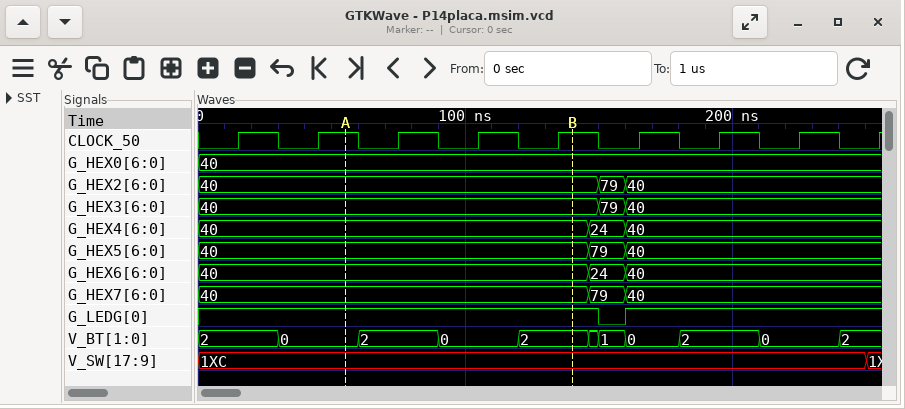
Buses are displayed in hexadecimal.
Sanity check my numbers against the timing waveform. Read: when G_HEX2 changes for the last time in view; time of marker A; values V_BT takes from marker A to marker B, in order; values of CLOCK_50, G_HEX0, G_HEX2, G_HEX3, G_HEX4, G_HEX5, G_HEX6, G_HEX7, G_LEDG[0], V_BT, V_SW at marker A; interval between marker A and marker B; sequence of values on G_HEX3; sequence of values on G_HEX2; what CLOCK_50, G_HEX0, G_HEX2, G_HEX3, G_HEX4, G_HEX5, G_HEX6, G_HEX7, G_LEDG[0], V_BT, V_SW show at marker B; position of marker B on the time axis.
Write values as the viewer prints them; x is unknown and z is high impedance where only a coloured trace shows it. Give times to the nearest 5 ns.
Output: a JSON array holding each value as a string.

["160 ns", "55 ns", "0, 2, 0, 2", "CLOCK_50=1, G_HEX0=40, G_HEX2=40, G_HEX3=40, G_HEX4=40, G_HEX5=40, G_HEX6=40, G_HEX7=40, G_LEDG[0]=1, V_BT=0, V_SW=1XC", "85 ns", "40, 79, 40", "40, 79, 40", "CLOCK_50=1, G_HEX0=40, G_HEX2=40, G_HEX3=40, G_HEX4=40, G_HEX5=40, G_HEX6=40, G_HEX7=40, G_LEDG[0]=1, V_BT=2, V_SW=1XC", "140 ns"]
